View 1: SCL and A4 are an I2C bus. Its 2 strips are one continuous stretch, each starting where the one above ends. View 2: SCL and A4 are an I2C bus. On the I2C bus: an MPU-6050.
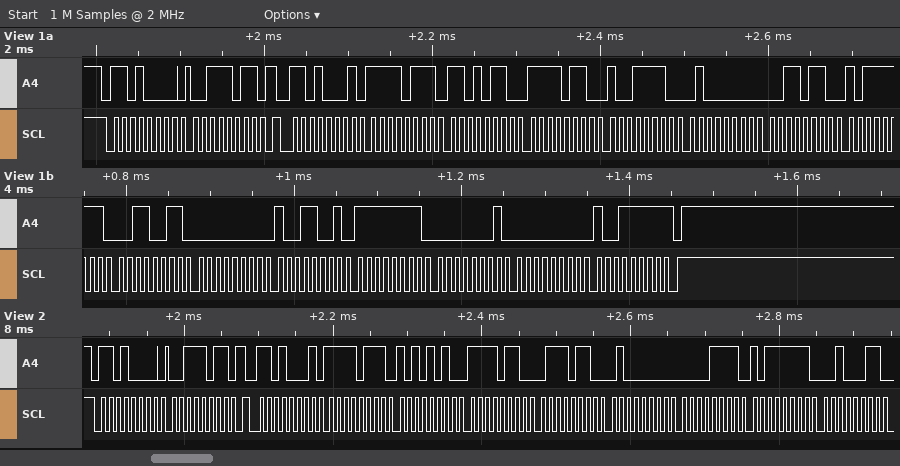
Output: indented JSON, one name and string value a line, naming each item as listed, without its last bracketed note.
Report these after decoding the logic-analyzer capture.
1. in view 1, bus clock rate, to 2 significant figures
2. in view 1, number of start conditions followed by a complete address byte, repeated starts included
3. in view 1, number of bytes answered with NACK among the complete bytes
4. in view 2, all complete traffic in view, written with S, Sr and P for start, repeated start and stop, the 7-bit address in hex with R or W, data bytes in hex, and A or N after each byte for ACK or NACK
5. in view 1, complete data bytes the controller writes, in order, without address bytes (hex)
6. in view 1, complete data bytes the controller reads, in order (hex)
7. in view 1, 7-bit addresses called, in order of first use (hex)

{
  "in view 1, bus clock rate, to 2 significant figures": "100 kHz",
  "in view 1, number of start conditions followed by a complete address byte, repeated starts included": "2",
  "in view 1, number of bytes answered with NACK among the complete bytes": "1",
  "in view 2, all complete traffic in view, written with S, Sr and P for start, repeated start and stop, the 7-bit address in hex with R or W, data bytes in hex, and A or N after each byte for ACK or NACK": "S 68W A 3B A Sr 68R A F7 A AA A F6 A 76 A 40 A 0F A BF A 23 A",
  "in view 1, complete data bytes the controller writes, in order, without address bytes": "3B",
  "in view 1, complete data bytes the controller reads, in order": "F7 D6 F6 9E 40 36 BF 33 00 99 FF 01 00 9F",
  "in view 1, 7-bit addresses called, in order of first use": "0x68"
}
